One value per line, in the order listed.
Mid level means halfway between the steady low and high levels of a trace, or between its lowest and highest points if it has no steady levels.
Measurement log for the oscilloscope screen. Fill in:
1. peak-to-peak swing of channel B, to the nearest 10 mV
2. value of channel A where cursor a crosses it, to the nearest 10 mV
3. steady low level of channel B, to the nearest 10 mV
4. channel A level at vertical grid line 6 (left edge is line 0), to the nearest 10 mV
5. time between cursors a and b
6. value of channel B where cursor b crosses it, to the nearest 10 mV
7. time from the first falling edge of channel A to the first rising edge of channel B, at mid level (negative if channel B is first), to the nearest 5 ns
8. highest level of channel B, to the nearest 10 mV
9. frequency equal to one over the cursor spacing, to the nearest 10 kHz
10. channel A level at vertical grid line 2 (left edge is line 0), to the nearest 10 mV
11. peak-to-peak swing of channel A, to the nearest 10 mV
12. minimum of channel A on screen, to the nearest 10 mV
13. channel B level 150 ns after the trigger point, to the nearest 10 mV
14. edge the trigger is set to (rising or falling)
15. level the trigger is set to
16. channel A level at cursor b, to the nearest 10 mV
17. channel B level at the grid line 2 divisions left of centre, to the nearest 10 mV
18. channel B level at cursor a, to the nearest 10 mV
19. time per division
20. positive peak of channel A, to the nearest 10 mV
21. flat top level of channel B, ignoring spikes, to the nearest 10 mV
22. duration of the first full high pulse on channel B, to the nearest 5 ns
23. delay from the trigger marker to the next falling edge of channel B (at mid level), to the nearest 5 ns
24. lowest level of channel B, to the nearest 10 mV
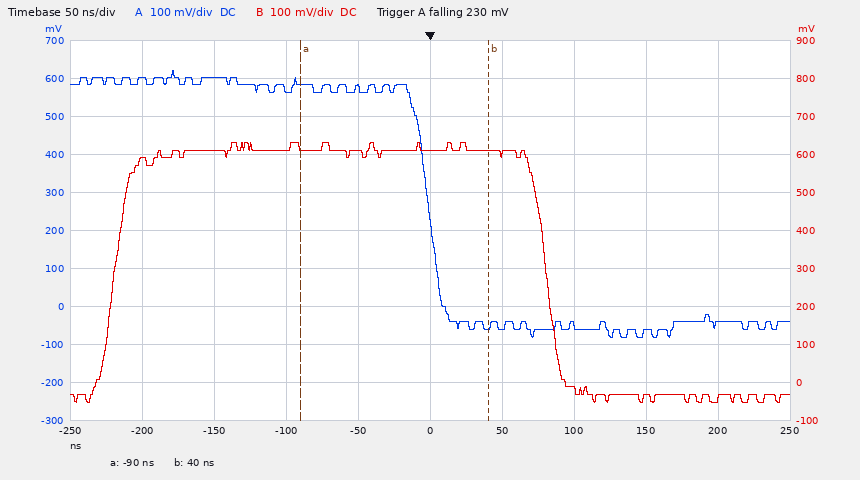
680 mV
580 mV
-30 mV
-50 mV
130 ns
610 mV
-220 ns
630 mV
7.69 MHz
600 mV
700 mV
-80 mV
-40 mV
falling
230 mV
-50 mV
610 mV
620 mV
50 ns
620 mV
610 mV
300 ns
80 ns
-50 mV
